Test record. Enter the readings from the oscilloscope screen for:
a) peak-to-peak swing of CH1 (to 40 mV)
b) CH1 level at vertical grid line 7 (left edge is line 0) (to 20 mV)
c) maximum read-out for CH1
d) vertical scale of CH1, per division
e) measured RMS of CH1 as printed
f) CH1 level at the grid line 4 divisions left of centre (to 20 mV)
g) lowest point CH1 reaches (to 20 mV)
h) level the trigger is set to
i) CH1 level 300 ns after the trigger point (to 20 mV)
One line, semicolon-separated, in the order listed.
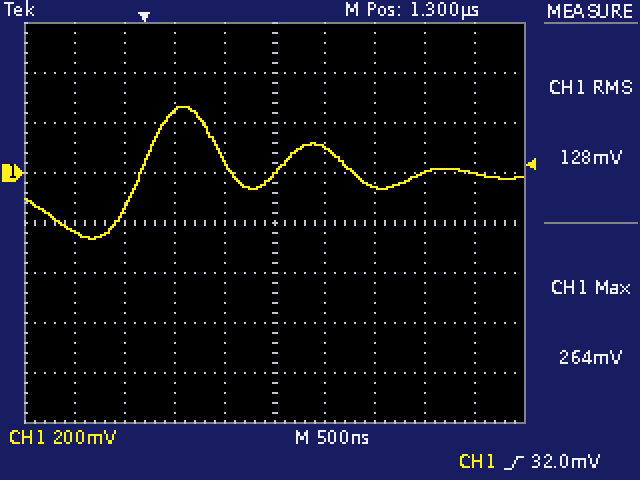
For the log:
520 mV; -60 mV; 264 mV; 200 mV; 128 mV; -240 mV; -260 mV; 32.0 mV; 240 mV
